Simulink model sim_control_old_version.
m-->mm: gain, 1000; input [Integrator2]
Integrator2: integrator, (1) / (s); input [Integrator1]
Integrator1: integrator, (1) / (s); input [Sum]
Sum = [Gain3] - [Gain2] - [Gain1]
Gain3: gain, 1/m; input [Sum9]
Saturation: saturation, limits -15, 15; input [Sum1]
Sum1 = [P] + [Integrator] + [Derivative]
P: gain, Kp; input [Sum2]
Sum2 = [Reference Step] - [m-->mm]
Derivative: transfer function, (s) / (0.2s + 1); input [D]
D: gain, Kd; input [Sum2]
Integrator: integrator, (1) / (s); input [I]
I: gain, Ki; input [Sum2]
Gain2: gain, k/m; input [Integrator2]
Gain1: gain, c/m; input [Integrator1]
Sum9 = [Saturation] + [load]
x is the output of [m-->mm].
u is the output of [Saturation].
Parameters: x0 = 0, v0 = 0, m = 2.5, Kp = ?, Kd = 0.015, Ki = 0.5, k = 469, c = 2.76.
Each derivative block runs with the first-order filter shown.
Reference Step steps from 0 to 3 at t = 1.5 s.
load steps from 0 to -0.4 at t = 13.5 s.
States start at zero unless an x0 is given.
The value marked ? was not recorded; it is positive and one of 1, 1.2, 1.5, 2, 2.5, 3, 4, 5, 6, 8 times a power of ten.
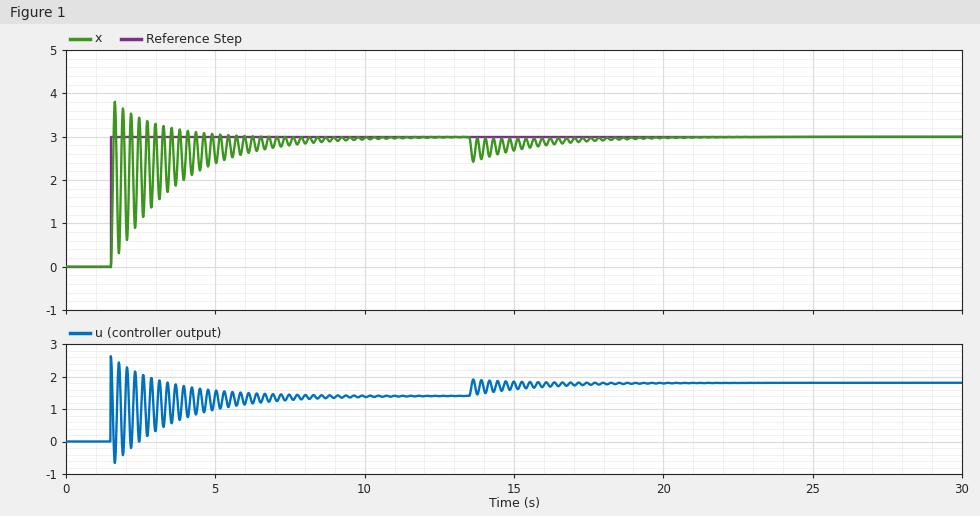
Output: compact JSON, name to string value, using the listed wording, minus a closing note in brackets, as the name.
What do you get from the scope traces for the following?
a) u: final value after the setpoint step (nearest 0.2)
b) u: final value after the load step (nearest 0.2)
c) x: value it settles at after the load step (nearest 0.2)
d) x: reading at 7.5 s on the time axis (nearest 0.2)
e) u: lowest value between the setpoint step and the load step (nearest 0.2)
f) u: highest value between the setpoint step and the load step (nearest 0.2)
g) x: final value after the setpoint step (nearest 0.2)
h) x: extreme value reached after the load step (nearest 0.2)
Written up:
{"u: final value after the setpoint step": "1.4", "u: final value after the load step": "1.8", "x: value it settles at after the load step": "3.0", "x: reading at 7.5 s on the time axis": "2.8", "u: lowest value between the setpoint step and the load step": "-0.6", "u: highest value between the setpoint step and the load step": "2.6", "x: final value after the setpoint step": "3.0", "x: extreme value reached after the load step": "2.4"}
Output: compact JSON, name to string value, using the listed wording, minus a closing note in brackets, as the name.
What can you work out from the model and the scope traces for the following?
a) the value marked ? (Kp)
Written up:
{"the value marked ?": "0.8"}
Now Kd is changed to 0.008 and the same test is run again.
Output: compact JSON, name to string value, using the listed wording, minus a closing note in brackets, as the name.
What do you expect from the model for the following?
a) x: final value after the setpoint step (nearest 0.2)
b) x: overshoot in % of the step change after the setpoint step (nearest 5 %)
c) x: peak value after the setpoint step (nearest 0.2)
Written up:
{"x: final value after the setpoint step": "3.0", "x: overshoot in % of the step change after the setpoint step": "25 %", "x: peak value after the setpoint step": "3.8"}
